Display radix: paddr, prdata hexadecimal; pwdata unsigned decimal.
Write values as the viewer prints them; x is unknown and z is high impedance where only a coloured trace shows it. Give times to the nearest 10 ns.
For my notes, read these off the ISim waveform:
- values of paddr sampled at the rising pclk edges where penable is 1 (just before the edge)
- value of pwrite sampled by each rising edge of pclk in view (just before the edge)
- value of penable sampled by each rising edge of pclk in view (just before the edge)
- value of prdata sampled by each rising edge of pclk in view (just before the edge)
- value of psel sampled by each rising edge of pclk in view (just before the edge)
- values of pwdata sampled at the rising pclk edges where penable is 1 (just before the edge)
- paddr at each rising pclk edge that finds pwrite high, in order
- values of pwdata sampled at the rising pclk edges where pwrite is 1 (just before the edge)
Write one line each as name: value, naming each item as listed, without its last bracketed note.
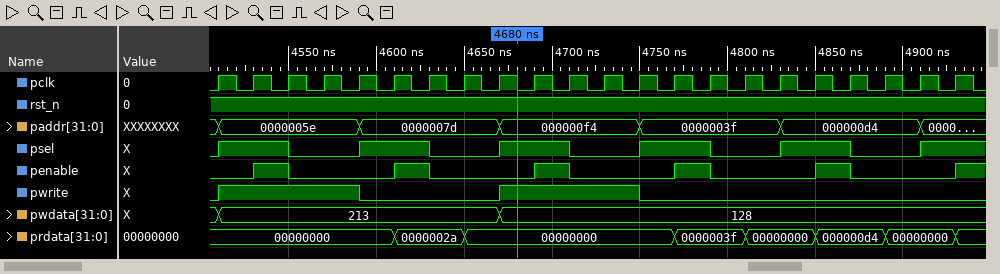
values of paddr sampled at the rising pclk edges where penable is 1: 0000005e, 0000007d, 000000f4, 0000003f, 000000d4
value of pwrite sampled by each rising edge of pclk in view: 0 1 1 1 1 0 0 0 0 1 1 1 1 0 0 0 0 0 0 0 0 0
value of penable sampled by each rising edge of pclk in view: 0 0 1 0 0 0 1 0 0 0 1 0 0 0 1 0 0 0 1 0 0 0
value of prdata sampled by each rising edge of pclk in view: 00000000, 00000000, 00000000, 00000000, 00000000, 00000000, 0000002a, 0000002a, 00000000, 00000000, 00000000, 00000000, 00000000, 00000000, 0000003f, 0000003f, 00000000, 00000000, 000000d4, 000000d4, 00000000, 00000000
value of psel sampled by each rising edge of pclk in view: 0 1 1 0 0 1 1 0 0 1 1 0 0 1 1 0 0 1 1 0 0 1
values of pwdata sampled at the rising pclk edges where penable is 1: 213, 213, 128, 128, 128
paddr at each rising pclk edge that finds pwrite high, in order: 0000005e, 0000005e, 0000005e, 0000005e, 000000f4, 000000f4, 000000f4, 000000f4
values of pwdata sampled at the rising pclk edges where pwrite is 1: 213, 213, 213, 213, 128, 128, 128, 128
